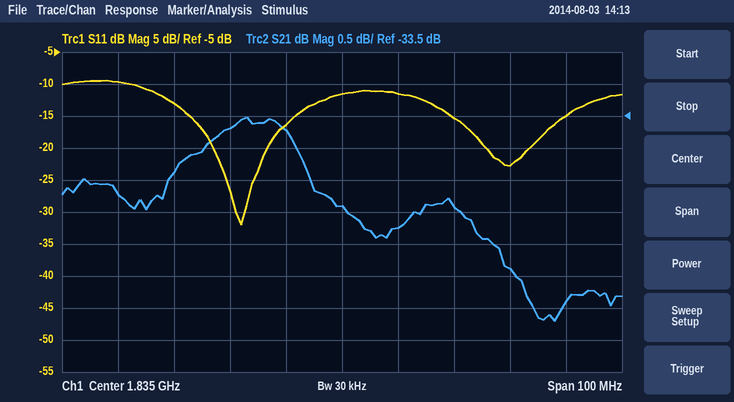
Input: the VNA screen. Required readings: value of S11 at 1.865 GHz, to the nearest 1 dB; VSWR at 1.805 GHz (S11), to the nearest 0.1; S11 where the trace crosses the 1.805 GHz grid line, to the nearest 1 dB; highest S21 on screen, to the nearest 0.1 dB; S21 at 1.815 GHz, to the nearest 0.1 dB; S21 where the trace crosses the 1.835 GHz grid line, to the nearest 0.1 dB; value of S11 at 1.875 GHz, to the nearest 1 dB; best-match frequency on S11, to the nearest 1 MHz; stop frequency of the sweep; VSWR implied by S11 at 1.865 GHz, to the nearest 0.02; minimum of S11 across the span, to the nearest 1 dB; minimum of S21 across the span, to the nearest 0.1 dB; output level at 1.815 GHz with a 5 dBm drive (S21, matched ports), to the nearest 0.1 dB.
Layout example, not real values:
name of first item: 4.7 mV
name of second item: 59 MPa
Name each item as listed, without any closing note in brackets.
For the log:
value of S11 at 1.865 GHz, to the nearest 1 dB: -23 dB
VSWR at 1.805 GHz (S11), to the nearest 0.1: 1.6
S11 where the trace crosses the 1.805 GHz grid line, to the nearest 1 dB: -13 dB
highest S21 on screen, to the nearest 0.1 dB: -33.5 dB
S21 at 1.815 GHz, to the nearest 0.1 dB: -33.7 dB
S21 where the trace crosses the 1.835 GHz grid line, to the nearest 0.1 dB: -34.9 dB
value of S11 at 1.875 GHz, to the nearest 1 dB: -15 dB
best-match frequency on S11, to the nearest 1 MHz: 1.817 GHz
stop frequency of the sweep: 1.885 GHz
VSWR implied by S11 at 1.865 GHz, to the nearest 0.02: 1.16
minimum of S11 across the span, to the nearest 1 dB: -32 dB
minimum of S21 across the span, to the nearest 0.1 dB: -36.7 dB
output level at 1.815 GHz with a 5 dBm drive (S21, matched ports), to the nearest 0.1 dB: -28.7 dBm
